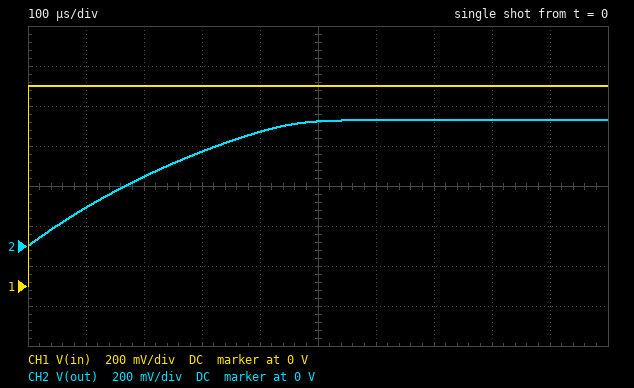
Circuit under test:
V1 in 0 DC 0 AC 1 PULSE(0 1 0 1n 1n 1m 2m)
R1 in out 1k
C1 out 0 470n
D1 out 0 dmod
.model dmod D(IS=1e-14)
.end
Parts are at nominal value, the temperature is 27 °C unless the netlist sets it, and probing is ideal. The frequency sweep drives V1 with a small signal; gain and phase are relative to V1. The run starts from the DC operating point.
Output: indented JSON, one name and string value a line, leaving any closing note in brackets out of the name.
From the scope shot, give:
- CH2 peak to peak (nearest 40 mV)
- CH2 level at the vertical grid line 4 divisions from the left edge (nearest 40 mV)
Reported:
{
  "CH2 peak to peak": "640 mV",
  "CH2 level at the vertical grid line 4 divisions from the left edge": "560 mV"
}
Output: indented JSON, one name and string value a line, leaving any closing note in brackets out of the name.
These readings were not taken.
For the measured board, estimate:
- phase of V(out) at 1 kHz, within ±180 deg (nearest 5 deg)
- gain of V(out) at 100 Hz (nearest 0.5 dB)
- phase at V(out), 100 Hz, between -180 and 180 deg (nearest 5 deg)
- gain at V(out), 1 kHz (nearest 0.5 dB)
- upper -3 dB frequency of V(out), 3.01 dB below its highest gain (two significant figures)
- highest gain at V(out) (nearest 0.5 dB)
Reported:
{
  "phase of V(out) at 1 kHz, within ±180 deg": "-70 deg",
  "gain of V(out) at 100 Hz": "-0.5 dB",
  "phase at V(out), 100 Hz, between -180 and 180 deg": "-15 deg",
  "gain at V(out), 1 kHz": "-10.0 dB",
  "upper -3 dB frequency of V(out), 3.01 dB below its highest gain": "340 Hz",
  "highest gain at V(out)": "0 dB"
}
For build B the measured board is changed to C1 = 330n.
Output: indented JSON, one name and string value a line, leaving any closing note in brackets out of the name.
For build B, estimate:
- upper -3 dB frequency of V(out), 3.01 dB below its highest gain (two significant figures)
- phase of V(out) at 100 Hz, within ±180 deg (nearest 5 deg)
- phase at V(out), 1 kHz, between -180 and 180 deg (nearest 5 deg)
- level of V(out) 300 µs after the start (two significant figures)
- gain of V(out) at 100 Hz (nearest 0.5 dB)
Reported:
{
  "upper -3 dB frequency of V(out), 3.01 dB below its highest gain": "480 Hz",
  "phase of V(out) at 100 Hz, within ±180 deg": "-10 deg",
  "phase at V(out), 1 kHz, between -180 and 180 deg": "-65 deg",
  "level of V(out) 300 µs after the start": "590 mV",
  "gain of V(out) at 100 Hz": "0 dB"
}
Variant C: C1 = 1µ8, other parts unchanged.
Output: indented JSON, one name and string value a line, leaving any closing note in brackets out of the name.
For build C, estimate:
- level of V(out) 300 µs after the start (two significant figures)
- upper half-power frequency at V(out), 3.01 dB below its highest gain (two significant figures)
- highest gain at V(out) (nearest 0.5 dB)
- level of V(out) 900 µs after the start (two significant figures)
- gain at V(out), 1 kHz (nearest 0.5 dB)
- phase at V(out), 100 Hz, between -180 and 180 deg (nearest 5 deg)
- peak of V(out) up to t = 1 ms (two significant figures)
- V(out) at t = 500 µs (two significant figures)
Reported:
{
  "level of V(out) 300 µs after the start": "150 mV",
  "upper half-power frequency at V(out), 3.01 dB below its highest gain": "88 Hz",
  "highest gain at V(out)": "0 dB",
  "level of V(out) 900 µs after the start": "390 mV",
  "gain at V(out), 1 kHz": "-21.0 dB",
  "phase at V(out), 100 Hz, between -180 and 180 deg": "-50 deg",
  "peak of V(out) up to t = 1 ms": "430 mV",
  "V(out) at t = 500 µs": "240 mV"
}
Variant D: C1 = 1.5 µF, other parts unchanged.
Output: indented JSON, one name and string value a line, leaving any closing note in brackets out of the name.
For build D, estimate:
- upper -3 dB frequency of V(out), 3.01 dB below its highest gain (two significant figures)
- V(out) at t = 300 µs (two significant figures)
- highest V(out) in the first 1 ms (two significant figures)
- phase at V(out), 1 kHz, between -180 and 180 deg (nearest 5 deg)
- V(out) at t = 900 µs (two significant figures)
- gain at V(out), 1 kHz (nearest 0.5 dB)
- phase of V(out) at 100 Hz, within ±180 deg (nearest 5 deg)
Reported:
{
  "upper -3 dB frequency of V(out), 3.01 dB below its highest gain": "110 Hz",
  "V(out) at t = 300 µs": "180 mV",
  "highest V(out) in the first 1 ms": "490 mV",
  "phase at V(out), 1 kHz, between -180 and 180 deg": "-85 deg",
  "V(out) at t = 900 µs": "450 mV",
  "gain at V(out), 1 kHz": "-19.5 dB",
  "phase of V(out) at 100 Hz, within ±180 deg": "-45 deg"
}
